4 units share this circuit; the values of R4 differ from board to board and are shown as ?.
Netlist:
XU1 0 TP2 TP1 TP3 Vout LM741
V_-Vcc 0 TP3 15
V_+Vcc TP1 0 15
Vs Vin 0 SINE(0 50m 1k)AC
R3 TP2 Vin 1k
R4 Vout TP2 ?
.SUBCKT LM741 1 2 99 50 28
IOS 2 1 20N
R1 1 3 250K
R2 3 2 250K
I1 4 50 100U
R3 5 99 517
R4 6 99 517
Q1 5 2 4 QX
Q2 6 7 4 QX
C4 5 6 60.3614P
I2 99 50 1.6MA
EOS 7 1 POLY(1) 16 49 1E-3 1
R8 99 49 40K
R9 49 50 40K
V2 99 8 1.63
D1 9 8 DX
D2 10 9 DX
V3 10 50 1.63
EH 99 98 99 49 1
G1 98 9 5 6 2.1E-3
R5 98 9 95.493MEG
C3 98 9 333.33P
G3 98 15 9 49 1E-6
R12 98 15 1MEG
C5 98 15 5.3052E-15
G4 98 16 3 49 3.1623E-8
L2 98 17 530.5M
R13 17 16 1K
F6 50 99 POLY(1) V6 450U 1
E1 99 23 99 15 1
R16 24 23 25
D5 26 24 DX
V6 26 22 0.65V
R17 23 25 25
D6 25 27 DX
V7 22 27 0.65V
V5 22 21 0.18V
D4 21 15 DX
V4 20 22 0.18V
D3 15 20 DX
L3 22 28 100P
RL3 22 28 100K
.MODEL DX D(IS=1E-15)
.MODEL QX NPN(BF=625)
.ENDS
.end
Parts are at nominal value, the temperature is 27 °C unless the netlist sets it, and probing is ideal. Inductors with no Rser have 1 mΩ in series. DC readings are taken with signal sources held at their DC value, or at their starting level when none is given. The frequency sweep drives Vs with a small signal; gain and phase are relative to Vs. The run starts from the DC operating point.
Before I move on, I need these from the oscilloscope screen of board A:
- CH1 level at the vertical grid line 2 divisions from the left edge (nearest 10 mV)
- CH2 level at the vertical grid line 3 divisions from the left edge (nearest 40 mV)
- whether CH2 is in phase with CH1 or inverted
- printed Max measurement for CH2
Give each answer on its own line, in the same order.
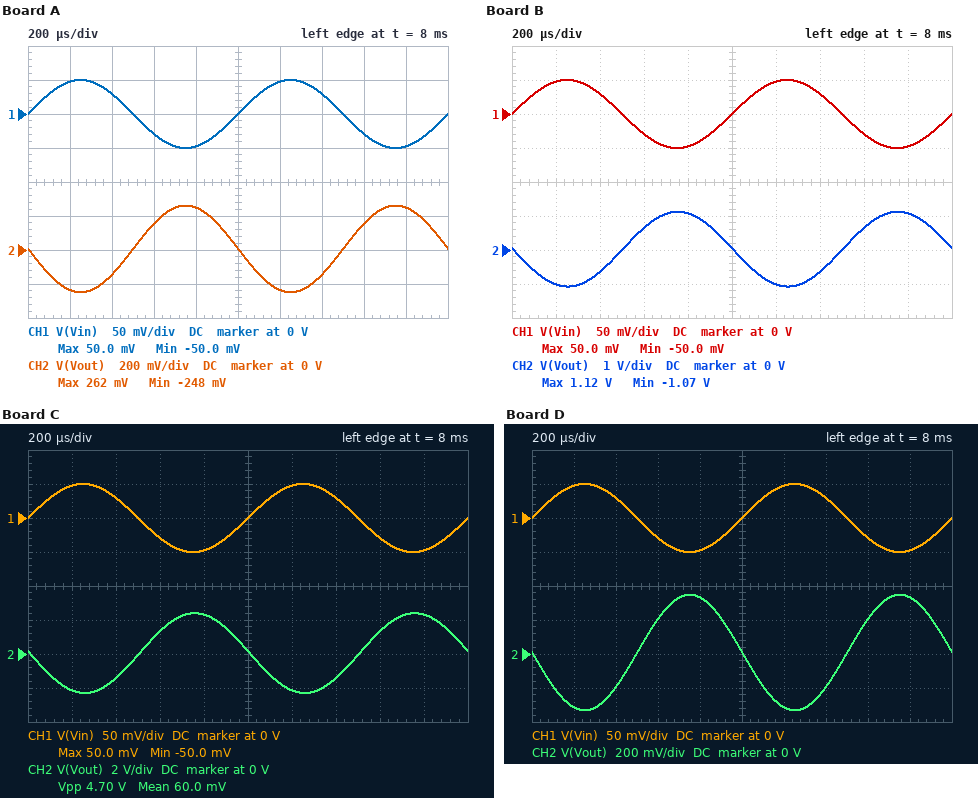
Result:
30 mV
160 mV
inverted
262 mV
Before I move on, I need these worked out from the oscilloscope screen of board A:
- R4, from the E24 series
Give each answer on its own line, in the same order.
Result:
5.1 kΩ
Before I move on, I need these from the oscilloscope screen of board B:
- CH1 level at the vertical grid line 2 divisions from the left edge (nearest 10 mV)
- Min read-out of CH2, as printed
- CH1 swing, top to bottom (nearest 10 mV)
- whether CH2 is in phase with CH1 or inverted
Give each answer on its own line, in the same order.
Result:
30 mV
-1.07 V
100 mV
inverted
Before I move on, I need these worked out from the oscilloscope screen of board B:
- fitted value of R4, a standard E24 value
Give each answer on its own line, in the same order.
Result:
22 kΩ
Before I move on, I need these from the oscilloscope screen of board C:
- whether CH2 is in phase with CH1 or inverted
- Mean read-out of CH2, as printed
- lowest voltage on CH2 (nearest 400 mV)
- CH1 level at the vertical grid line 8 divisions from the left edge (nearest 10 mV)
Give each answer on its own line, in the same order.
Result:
inverted
60.0 mV
-2.4 V
-30 mV
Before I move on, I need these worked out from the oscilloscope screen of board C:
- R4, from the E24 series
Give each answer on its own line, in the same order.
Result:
47 kΩ
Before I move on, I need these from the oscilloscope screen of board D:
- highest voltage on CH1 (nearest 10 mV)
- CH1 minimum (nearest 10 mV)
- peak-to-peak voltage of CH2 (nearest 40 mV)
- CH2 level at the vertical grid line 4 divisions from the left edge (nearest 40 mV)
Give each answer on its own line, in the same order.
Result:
50 mV
-50 mV
680 mV
320 mV
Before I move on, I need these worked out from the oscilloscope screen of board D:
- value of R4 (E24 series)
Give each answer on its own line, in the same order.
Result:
6.8 kΩ
